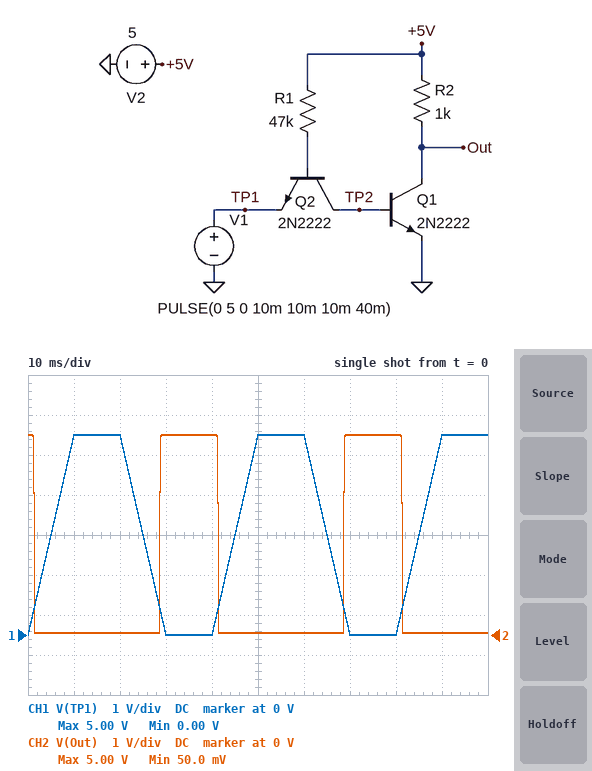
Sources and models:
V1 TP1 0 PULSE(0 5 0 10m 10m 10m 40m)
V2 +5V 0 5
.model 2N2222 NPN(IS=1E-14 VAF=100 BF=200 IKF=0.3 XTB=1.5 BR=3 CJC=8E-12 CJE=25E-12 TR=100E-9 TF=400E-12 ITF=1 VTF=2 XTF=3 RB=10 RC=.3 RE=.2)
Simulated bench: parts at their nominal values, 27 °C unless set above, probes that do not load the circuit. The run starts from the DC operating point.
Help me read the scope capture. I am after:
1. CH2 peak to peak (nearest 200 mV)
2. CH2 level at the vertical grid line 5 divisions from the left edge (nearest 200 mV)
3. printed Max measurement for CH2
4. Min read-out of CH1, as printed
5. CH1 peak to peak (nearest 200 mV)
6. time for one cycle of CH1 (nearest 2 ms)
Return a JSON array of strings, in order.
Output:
["5.0 V", "0 V", "5.00 V", "0.00 V", "5.0 V", "40 ms"]
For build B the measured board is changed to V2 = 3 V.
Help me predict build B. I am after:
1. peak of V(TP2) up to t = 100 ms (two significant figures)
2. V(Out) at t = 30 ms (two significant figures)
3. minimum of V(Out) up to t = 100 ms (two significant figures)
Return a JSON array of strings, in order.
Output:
["690 mV", "3.0 V", "59 mV"]
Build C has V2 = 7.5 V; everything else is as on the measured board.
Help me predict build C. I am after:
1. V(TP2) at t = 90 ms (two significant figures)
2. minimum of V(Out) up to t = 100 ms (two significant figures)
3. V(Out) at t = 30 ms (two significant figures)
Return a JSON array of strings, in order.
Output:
["720 mV", "53 mV", "7.5 V"]
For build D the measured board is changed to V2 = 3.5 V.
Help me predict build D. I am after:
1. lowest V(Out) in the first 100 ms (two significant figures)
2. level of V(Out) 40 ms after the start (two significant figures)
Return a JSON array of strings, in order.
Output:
["57 mV", "3.5 V"]
